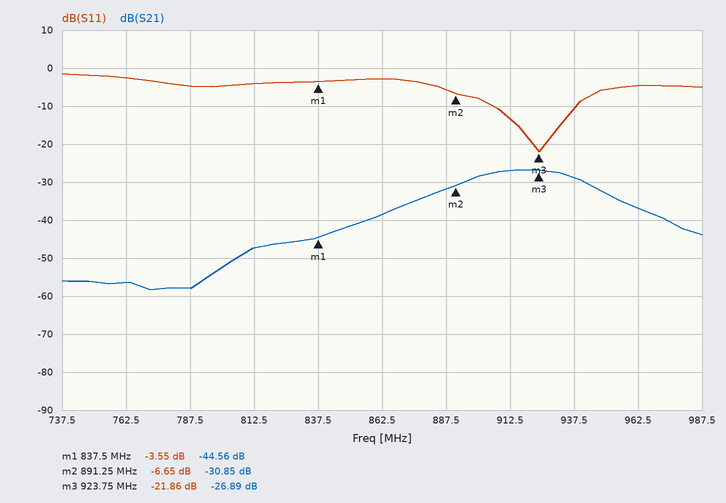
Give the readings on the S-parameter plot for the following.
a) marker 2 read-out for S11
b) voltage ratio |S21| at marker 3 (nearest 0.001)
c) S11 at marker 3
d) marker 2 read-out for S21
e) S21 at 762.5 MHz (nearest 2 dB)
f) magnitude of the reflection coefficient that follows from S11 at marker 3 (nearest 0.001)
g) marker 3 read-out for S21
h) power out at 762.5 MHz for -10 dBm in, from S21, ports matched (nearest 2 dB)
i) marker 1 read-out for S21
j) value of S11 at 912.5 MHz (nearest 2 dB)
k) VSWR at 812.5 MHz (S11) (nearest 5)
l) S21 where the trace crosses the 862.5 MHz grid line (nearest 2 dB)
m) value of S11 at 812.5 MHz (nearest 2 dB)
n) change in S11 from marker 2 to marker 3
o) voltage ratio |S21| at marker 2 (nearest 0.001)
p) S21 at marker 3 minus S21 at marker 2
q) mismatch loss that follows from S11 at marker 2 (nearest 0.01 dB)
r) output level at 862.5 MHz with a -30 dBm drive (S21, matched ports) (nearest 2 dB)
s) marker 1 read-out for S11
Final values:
-6.65 dB
0.045
-21.86 dB
-30.85 dB
-56 dB
0.081
-26.89 dB
-66 dBm
-44.56 dB
-14 dB
5
-38 dB
-4 dB
-15.21 dB
0.029
3.96 dB
1.06 dB
-68 dBm
-3.55 dB
